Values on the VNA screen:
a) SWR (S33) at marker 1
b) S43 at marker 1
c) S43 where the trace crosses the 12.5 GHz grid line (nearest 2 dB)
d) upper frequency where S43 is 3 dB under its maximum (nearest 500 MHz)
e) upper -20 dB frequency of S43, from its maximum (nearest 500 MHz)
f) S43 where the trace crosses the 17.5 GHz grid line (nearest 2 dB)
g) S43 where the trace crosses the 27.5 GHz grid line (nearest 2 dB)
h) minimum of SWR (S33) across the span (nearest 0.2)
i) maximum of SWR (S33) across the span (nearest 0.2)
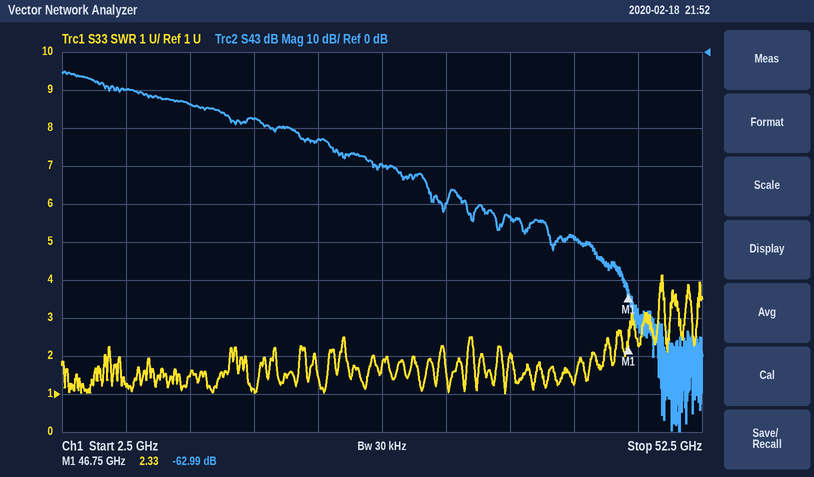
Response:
2.33
-62.99 dB
-14 dB
5.5 GHz
23.5 GHz
-18 dB
-30 dB
1.0
4.2
